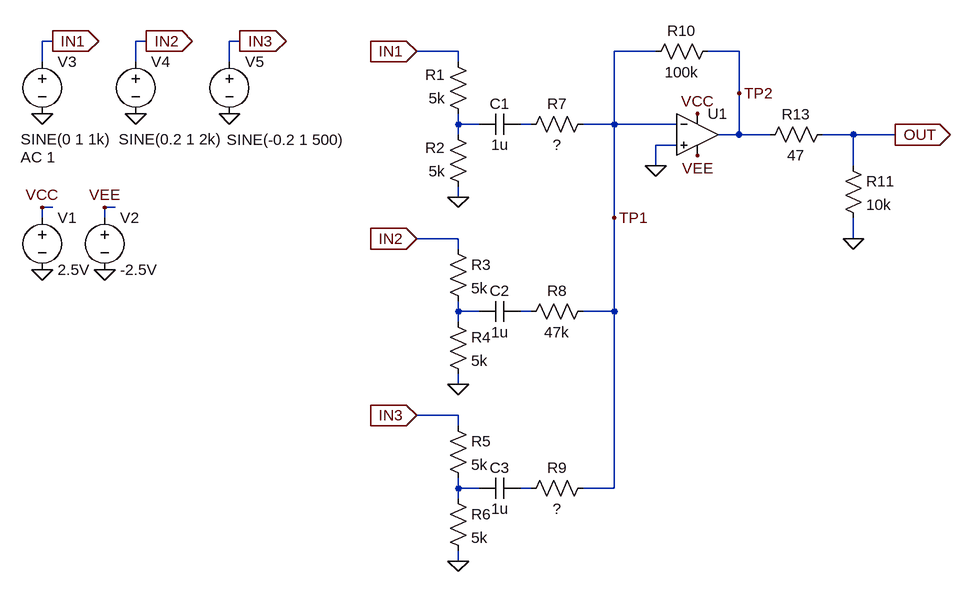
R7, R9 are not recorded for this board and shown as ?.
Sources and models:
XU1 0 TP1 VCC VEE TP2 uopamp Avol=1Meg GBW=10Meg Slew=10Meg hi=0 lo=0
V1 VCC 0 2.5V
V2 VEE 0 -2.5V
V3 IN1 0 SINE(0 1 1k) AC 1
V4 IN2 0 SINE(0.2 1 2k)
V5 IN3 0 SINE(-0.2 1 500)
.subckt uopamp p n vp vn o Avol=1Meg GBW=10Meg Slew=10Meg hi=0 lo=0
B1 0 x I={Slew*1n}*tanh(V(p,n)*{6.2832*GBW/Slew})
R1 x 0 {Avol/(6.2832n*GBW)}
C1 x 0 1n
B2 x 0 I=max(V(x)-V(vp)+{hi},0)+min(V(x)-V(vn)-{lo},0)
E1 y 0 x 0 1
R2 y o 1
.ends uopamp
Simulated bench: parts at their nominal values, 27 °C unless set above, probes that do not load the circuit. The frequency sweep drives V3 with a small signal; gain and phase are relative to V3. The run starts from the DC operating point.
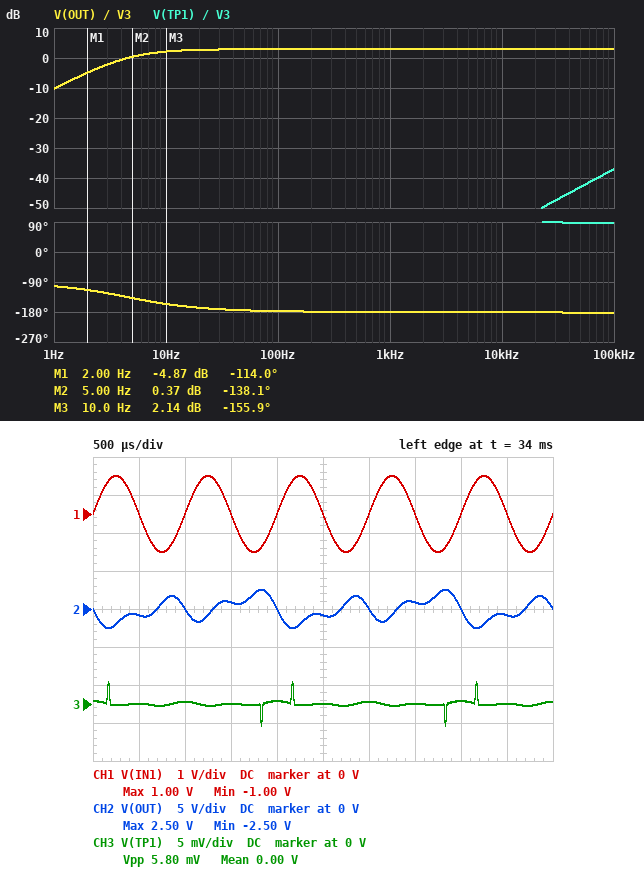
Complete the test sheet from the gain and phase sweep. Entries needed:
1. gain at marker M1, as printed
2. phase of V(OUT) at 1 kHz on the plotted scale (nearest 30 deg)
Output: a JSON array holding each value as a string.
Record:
["-4.87 dB", "-180 deg"]
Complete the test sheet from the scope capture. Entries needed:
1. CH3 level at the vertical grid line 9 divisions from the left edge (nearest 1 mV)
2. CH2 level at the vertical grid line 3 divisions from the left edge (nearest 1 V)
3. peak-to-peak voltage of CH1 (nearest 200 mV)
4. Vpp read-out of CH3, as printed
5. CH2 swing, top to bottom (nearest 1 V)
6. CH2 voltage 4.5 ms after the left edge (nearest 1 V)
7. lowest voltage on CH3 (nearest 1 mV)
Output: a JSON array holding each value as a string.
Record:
["0 V", "1 V", "2.0 V", "5.80 mV", "5 V", "-1 V", "-3 mV"]
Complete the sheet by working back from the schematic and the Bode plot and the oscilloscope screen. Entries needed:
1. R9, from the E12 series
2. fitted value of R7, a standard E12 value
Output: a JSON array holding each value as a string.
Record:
["56 kΩ", "33 kΩ"]
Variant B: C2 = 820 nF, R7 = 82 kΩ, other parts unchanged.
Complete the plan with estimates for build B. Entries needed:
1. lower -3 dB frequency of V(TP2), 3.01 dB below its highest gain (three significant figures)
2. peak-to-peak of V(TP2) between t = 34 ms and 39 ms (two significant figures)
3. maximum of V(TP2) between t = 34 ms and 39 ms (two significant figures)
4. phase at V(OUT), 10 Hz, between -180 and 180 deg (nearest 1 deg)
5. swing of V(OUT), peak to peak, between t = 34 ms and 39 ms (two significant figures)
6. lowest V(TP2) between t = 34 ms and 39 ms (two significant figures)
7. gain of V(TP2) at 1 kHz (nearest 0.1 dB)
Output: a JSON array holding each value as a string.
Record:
["1.88 Hz", "3.7 V", "1.8 V", "-169 deg", "3.6 V", "-1.8 V", "-4.6 dB"]
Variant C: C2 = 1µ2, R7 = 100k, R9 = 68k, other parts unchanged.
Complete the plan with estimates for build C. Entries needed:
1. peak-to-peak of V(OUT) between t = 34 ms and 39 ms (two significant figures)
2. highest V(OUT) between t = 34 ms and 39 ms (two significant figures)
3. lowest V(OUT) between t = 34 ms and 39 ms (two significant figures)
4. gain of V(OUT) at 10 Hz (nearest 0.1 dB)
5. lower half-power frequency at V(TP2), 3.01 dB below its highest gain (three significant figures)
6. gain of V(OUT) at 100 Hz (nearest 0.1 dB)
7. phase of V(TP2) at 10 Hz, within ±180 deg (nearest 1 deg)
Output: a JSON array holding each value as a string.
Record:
["3.3 V", "1.7 V", "-1.7 V", "-6.4 dB", "1.55 Hz", "-6.3 dB", "-171 deg"]
